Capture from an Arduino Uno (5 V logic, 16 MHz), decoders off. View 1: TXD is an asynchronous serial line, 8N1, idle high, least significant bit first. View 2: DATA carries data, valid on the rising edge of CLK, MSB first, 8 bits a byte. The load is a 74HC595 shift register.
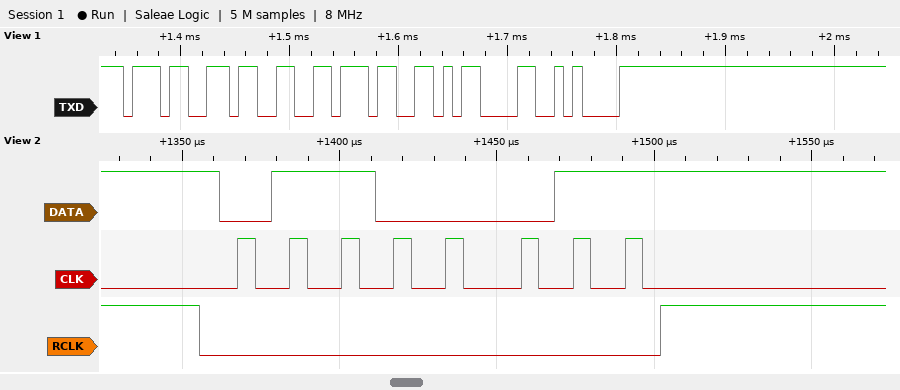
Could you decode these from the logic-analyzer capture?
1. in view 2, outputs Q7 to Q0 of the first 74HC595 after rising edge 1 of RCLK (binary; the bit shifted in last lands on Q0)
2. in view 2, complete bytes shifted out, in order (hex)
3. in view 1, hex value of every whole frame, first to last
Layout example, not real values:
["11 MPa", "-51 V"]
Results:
["01100011", "63", "37 33 37 0D 0A"]
